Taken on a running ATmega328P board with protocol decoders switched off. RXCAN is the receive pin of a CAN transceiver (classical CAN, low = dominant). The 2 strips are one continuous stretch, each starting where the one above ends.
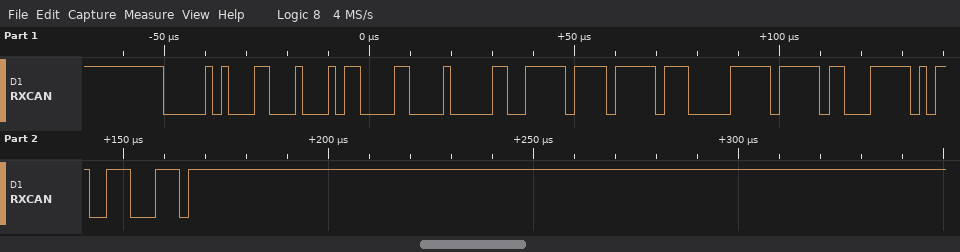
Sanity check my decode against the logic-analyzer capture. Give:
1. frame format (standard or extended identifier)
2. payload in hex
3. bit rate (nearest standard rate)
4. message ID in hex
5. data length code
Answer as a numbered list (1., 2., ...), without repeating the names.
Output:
1. standard
2. B0 C2 09 FF 7F 83 FF 8F
3. 500 kbit/s
4. 0x023
5. 8
